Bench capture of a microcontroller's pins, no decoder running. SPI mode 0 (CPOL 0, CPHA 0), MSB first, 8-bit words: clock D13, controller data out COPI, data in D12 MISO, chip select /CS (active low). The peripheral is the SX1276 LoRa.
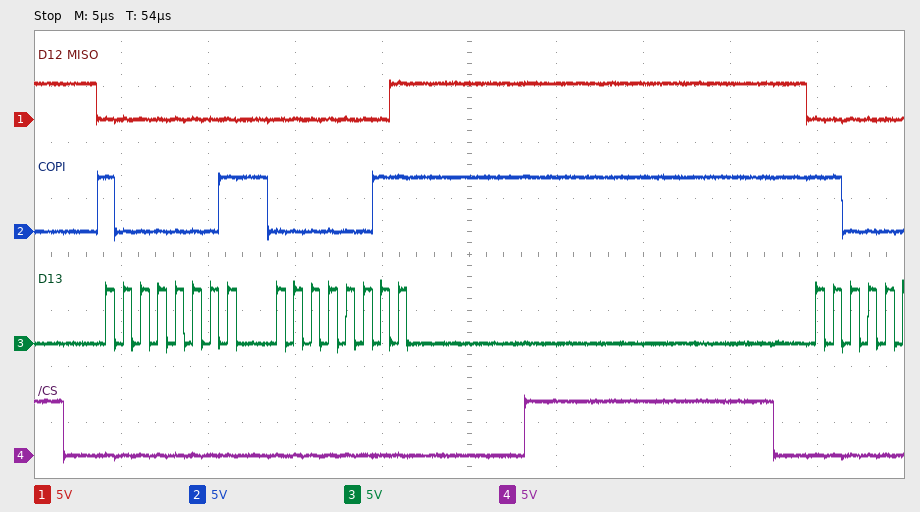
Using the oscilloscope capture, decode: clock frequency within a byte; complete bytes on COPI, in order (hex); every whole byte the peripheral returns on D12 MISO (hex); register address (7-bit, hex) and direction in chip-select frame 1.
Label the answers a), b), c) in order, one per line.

a) 1 MHz
b) 0x81 0x03
c) 0x00 0x01
d) 0x01 write
